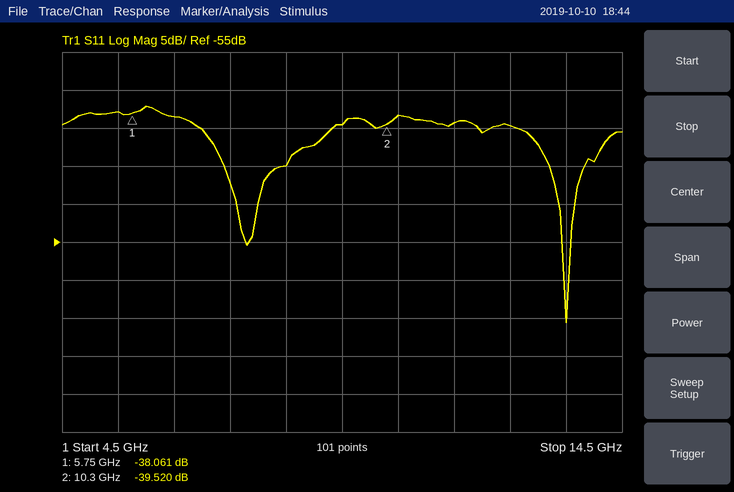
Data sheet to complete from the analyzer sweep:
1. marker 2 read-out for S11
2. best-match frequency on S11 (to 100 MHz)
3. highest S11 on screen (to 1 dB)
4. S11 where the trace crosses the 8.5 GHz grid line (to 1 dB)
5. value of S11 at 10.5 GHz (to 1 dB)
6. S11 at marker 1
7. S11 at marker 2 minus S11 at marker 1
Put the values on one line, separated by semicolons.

-39.520 dB; 13.5 GHz; -37 dB; -45 dB; -38 dB; -38.061 dB; -1.459 dB
